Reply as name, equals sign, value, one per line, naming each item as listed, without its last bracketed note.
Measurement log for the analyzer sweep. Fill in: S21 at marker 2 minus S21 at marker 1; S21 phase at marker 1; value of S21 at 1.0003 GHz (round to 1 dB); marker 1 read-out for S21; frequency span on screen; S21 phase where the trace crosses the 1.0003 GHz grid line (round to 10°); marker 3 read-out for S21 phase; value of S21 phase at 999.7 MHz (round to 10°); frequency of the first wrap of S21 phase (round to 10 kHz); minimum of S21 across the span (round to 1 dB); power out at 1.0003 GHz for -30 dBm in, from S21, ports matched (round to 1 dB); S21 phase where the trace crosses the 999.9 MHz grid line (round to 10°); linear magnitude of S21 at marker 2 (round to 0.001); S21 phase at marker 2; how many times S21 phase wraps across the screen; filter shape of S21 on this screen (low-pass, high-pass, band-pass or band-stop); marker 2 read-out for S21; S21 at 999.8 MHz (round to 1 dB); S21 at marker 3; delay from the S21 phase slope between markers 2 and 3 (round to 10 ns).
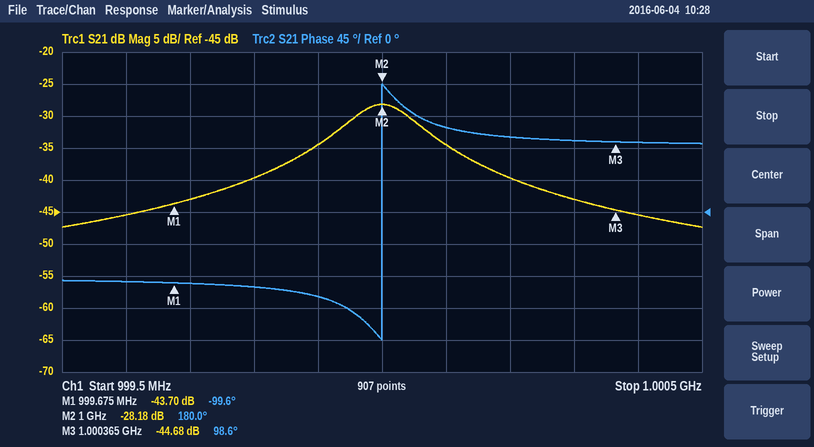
S21 at marker 2 minus S21 at marker 1 = 15.52 dB
S21 phase at marker 1 = -99.6°
value of S21 at 1.0003 GHz = -43 dB
marker 1 read-out for S21 = -43.70 dB
frequency span on screen = 1 MHz
S21 phase where the trace crosses the 1.0003 GHz grid line = 100°
marker 3 read-out for S21 phase = 98.6°
value of S21 phase at 999.7 MHz = -100°
frequency of the first wrap of S21 phase = 1.00000 GHz
minimum of S21 across the span = -47 dB
power out at 1.0003 GHz for -30 dBm in, from S21, ports matched = -73 dBm
S21 phase where the trace crosses the 999.9 MHz grid line = -120°
linear magnitude of S21 at marker 2 = 0.039
S21 phase at marker 2 = 180.0°
how many times S21 phase wraps across the screen = 1
filter shape of S21 on this screen = band-pass
marker 2 read-out for S21 = -28.18 dB
S21 at 999.8 MHz = -40 dB
S21 at marker 3 = -44.68 dB
delay from the S21 phase slope between markers 2 and 3 = 620 ns
